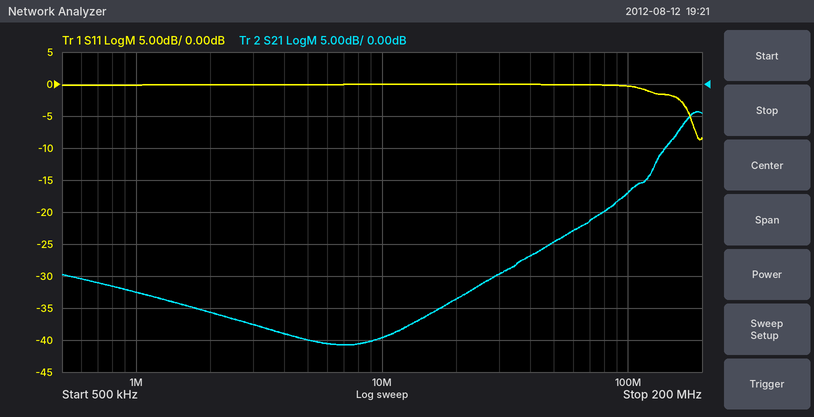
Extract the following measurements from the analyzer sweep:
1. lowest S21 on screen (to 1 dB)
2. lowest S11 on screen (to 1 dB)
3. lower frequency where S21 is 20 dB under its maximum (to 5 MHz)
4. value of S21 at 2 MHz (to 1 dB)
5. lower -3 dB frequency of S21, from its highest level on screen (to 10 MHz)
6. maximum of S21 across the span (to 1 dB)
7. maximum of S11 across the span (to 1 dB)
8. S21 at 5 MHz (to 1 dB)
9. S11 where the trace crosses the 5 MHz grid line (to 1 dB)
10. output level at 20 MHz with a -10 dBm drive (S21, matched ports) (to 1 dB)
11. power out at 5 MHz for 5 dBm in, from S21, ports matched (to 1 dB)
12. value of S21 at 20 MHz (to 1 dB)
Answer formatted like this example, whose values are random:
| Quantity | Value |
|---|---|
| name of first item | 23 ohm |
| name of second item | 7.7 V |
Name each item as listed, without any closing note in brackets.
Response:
| Quantity | Value |
|---|---|
| lowest S21 on screen | -41 dB |
| lowest S11 on screen | -9 dB |
| lower frequency where S21 is 20 dB under its maximum | 50 MHz |
| value of S21 at 2 MHz | -36 dB |
| lower -3 dB frequency of S21, from its highest level on screen | 160 MHz |
| maximum of S21 across the span | -4 dB |
| maximum of S11 across the span | 0 dB |
| S21 at 5 MHz | -40 dB |
| S11 where the trace crosses the 5 MHz grid line | 0 dB |
| output level at 20 MHz with a -10 dBm drive (S21, matched ports) | -44 dBm |
| power out at 5 MHz for 5 dBm in, from S21, ports matched | -35 dBm |
| value of S21 at 20 MHz | -34 dB |
